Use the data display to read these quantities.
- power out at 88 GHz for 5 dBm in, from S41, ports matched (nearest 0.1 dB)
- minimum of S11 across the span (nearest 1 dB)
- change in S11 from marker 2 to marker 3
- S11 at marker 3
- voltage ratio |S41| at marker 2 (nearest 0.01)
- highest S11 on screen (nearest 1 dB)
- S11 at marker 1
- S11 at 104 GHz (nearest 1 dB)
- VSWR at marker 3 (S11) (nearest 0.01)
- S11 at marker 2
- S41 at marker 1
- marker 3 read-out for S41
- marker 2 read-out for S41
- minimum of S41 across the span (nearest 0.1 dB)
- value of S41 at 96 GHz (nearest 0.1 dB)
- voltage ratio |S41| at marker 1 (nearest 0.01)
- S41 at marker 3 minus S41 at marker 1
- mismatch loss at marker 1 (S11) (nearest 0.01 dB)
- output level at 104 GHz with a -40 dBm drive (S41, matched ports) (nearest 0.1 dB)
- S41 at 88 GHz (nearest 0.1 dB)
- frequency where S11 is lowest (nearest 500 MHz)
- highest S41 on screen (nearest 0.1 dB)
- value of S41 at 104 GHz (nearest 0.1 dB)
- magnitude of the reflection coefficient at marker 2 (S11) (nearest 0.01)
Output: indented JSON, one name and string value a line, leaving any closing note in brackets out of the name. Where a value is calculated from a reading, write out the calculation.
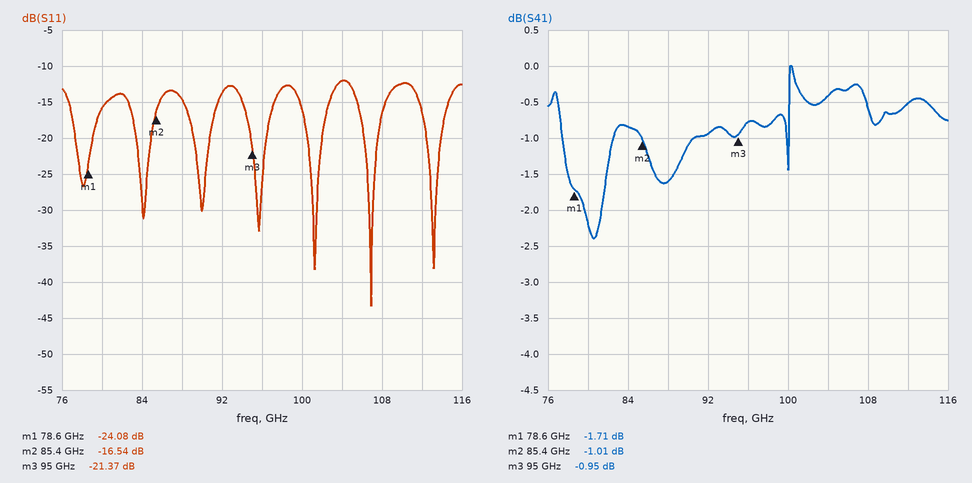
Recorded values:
{
  "power out at 88 GHz for 5 dBm in, from S41, ports matched": "5 dBm + (-1.6 dB) = 3.4 dBm",
  "minimum of S11 across the span": "-43 dB",
  "change in S11 from marker 2 to marker 3": "-21.37 − (-16.54) = -4.83 dB",
  "S11 at marker 3": "-21.37 dB",
  "voltage ratio |S41| at marker 2": "10^(-1.01/20) ≈ 0.89",
  "highest S11 on screen": "-12 dB",
  "S11 at marker 1": "-24.08 dB",
  "S11 at 104 GHz": "-12 dB",
  "VSWR at marker 3 (S11)": "(1 + 0.0854)/(1 − 0.0854) ≈ 1.19",
  "S11 at marker 2": "-16.54 dB",
  "S41 at marker 1": "-1.71 dB",
  "marker 3 read-out for S41": "-0.95 dB",
  "marker 2 read-out for S41": "-1.01 dB",
  "minimum of S41 across the span": "-2.4 dB",
  "value of S41 at 96 GHz": "-0.8 dB",
  "voltage ratio |S41| at marker 1": "10^(-1.71/20) ≈ 0.82",
  "S41 at marker 3 minus S41 at marker 1": "-0.95 − (-1.71) = 0.76 dB",
  "mismatch loss at marker 1 (S11)": "−10 log10(1 − 10^(-24.08/10)) ≈ 0.02 dB",
  "output level at 104 GHz with a -40 dBm drive (S41, matched ports)": "-40 dBm + (-0.4 dB) = -40.4 dBm",
  "S41 at 88 GHz": "-1.6 dB",
  "frequency where S11 is lowest": "107.0 GHz",
  "highest S41 on screen": "0.0 dB",
  "value of S41 at 104 GHz": "-0.4 dB",
  "magnitude of the reflection coefficient at marker 2 (S11)": "10^(-16.54/20) ≈ 0.15"
}
